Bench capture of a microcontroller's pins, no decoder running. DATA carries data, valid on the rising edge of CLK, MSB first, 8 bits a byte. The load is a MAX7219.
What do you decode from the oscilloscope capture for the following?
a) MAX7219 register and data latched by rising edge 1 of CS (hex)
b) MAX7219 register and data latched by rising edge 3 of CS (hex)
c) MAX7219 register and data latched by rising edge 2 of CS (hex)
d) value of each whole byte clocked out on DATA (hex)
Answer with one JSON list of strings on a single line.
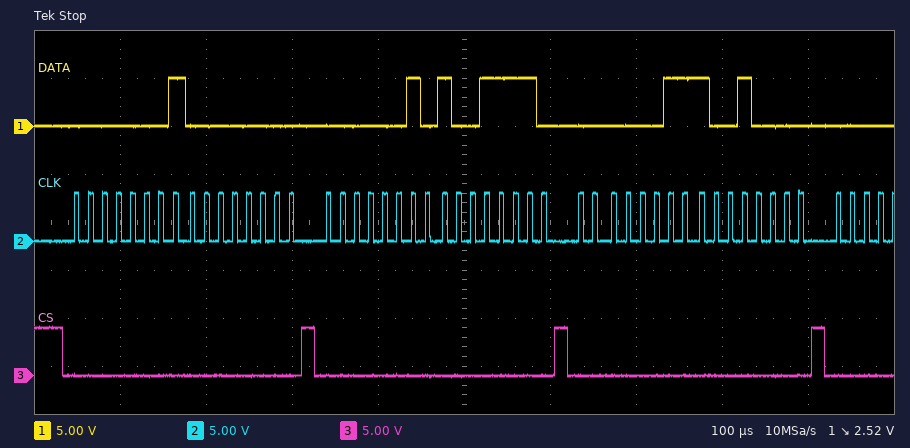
["register 0x1, data 0x00", "register 0x3, data 0x90", "register 0x2, data 0x9E", "01 00 02 9E 03 90"]
